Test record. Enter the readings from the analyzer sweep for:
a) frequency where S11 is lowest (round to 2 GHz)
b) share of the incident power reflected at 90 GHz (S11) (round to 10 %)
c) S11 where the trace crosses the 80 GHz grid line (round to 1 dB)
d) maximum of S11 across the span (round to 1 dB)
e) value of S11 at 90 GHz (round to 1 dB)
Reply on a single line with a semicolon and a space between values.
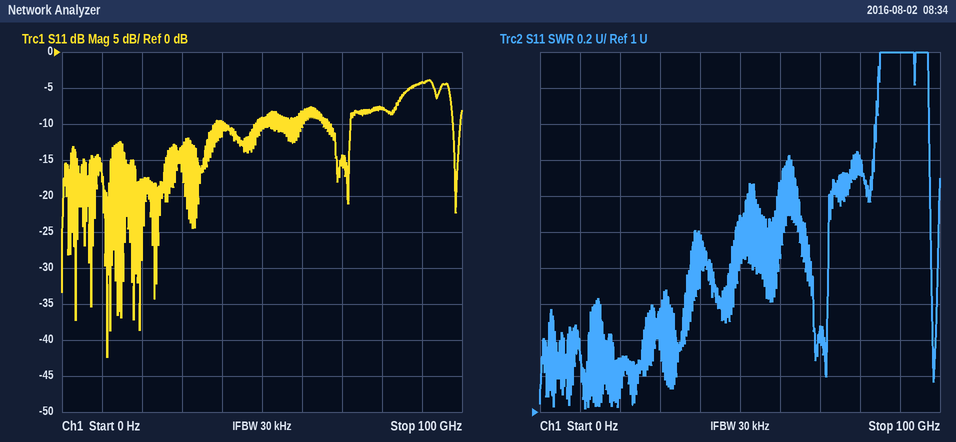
12 GHz; 40 %; -8 dB; -4 dB; -4 dB
